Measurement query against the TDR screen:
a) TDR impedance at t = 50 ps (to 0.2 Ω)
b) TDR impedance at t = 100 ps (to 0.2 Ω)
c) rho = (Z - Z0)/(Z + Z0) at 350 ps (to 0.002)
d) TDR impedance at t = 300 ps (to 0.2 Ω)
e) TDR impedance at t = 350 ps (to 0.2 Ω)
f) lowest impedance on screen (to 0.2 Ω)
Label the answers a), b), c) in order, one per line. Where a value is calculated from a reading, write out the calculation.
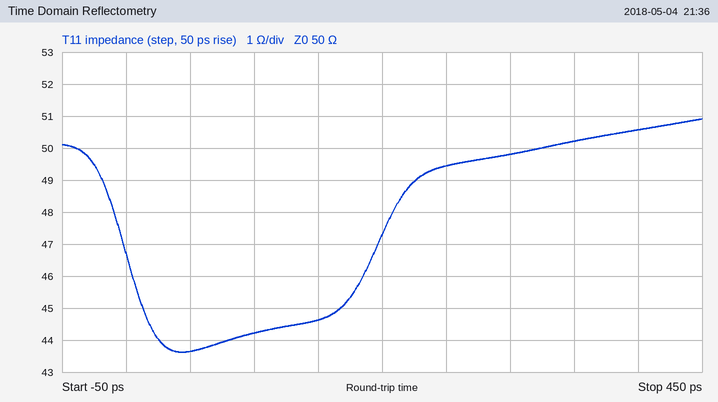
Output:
a) 43.6 Ω
b) 44.2 Ω
c) (50.2 − 50)/(50.2 + 50) ≈ +0.002
d) 49.8 Ω
e) 50.2 Ω
f) 43.6 Ω
